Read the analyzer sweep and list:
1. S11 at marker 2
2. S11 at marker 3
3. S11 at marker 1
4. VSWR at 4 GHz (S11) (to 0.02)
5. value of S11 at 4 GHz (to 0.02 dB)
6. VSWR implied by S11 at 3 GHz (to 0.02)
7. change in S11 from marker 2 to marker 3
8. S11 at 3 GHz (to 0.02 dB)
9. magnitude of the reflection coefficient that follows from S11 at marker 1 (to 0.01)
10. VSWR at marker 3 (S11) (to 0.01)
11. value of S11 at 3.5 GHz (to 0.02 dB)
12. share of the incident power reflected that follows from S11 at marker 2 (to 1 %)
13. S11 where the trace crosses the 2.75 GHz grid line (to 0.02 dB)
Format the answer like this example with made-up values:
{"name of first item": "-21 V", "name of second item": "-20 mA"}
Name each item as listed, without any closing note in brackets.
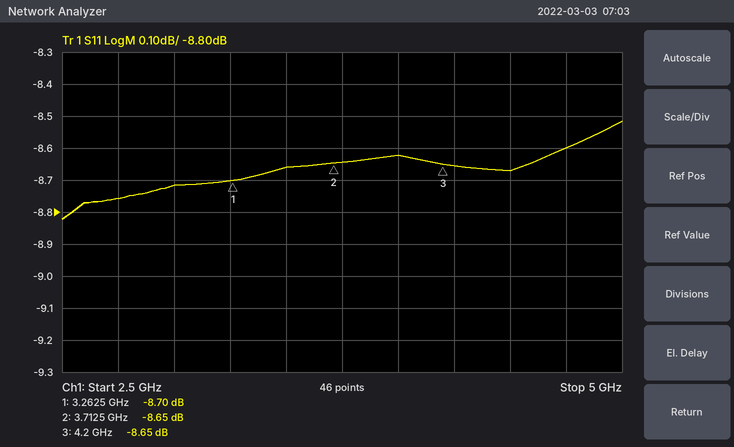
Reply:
{"S11 at marker 2": "-8.65 dB", "S11 at marker 3": "-8.65 dB", "S11 at marker 1": "-8.70 dB", "VSWR at 4 GHz (S11)": "2.18", "value of S11 at 4 GHz": "-8.62 dB", "VSWR implied by S11 at 3 GHz": "2.16", "change in S11 from marker 2 to marker 3": "0.00 dB", "S11 at 3 GHz": "-8.72 dB", "magnitude of the reflection coefficient that follows from S11 at marker 1": "0.37", "VSWR at marker 3 (S11)": "2.17", "value of S11 at 3.5 GHz": "-8.66 dB", "share of the incident power reflected that follows from S11 at marker 2": "14 %", "S11 where the trace crosses the 2.75 GHz grid line": "-8.76 dB"}
